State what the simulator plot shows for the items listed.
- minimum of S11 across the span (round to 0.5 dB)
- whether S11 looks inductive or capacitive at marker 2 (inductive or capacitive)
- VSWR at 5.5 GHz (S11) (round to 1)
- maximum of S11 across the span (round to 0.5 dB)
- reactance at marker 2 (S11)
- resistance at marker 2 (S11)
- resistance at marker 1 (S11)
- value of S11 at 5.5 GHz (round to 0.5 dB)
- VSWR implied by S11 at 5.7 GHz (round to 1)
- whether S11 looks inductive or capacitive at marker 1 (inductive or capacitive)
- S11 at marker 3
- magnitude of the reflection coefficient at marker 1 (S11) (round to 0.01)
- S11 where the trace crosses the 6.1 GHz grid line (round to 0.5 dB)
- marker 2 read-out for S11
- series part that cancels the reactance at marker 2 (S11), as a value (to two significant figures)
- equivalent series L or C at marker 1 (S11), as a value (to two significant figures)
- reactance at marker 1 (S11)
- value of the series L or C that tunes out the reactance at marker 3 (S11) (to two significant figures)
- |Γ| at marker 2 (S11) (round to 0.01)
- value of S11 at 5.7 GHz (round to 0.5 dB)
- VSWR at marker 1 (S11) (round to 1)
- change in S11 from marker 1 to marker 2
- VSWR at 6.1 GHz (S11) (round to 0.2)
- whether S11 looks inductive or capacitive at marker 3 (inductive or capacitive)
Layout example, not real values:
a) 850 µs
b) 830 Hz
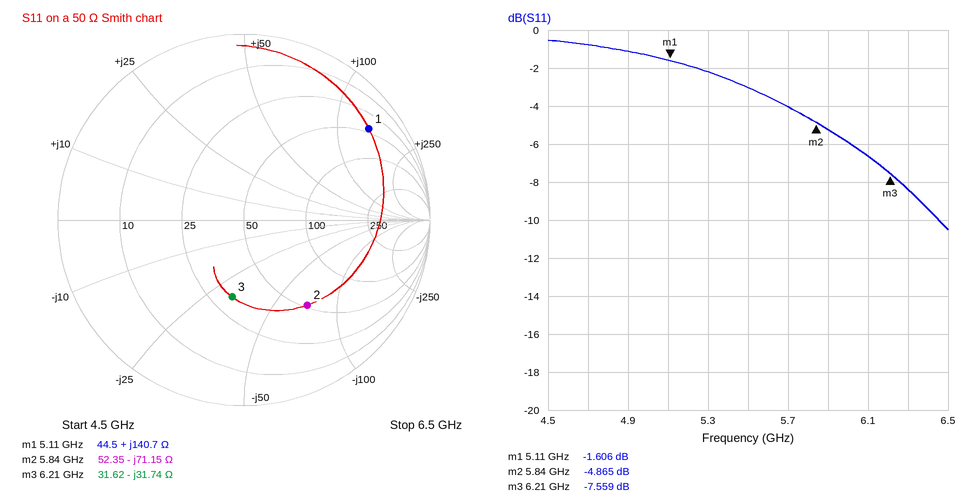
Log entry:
a) -10.5 dB
b) capacitive
c) 6
d) -0.5 dB
e) -71.15 Ω
f) 52.35 Ω
g) 44.5 Ω
h) -3.0 dB
i) 4
j) inductive
k) -7.559 dB
l) 0.83
m) -6.5 dB
n) -4.865 dB
o) 1.9 nH
p) 4.4 nH
q) +140.7 Ω
r) 810 pH
s) 0.57
t) -4.0 dB
u) 11
v) -3.259 dB
w) 2.8
x) capacitive
